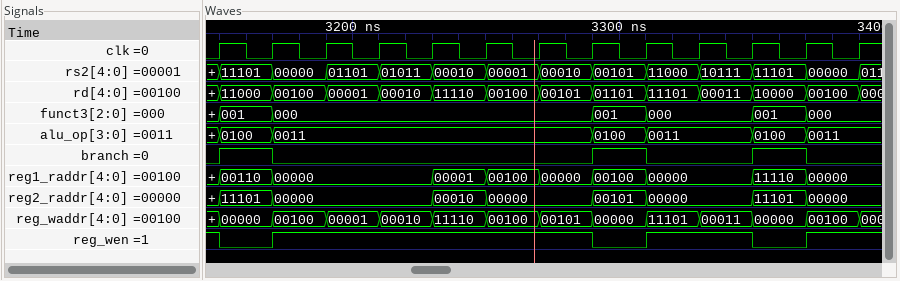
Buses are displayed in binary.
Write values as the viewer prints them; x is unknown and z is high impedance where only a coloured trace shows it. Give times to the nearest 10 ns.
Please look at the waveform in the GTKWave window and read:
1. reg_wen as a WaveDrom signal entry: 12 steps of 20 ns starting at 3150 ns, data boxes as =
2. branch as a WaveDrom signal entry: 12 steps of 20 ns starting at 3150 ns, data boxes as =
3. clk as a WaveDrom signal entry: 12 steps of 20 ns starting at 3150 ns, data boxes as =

{name: 'reg_wen', wave: '01.....01.01'}
{name: 'branch', wave: '10.....10.10'}
{name: 'clk', wave: 'p...........'}
